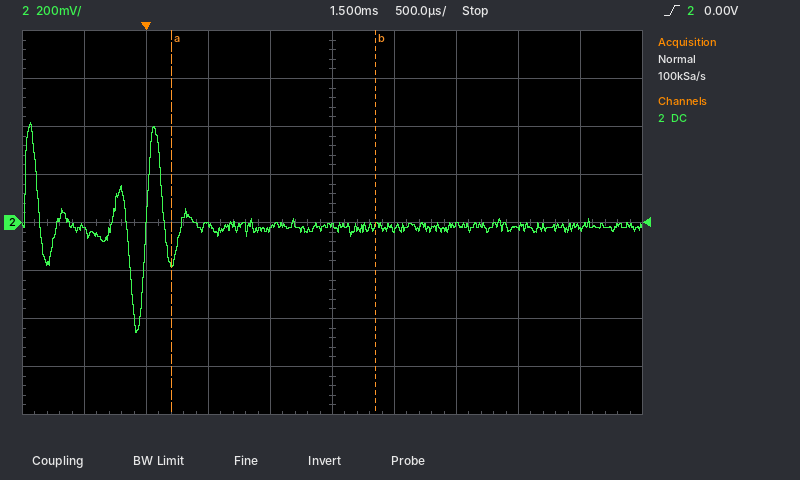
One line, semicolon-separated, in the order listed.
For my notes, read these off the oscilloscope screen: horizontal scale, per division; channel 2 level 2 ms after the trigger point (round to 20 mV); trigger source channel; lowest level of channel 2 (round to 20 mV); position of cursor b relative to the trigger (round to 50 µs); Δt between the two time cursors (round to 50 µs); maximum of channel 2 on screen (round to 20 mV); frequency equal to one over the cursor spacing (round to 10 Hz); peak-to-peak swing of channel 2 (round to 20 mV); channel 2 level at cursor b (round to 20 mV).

500 µs; -20 mV; channel 2; -460 mV; +1.85 ms; 1.65 ms; 420 mV; 610 Hz; 880 mV; -20 mV
